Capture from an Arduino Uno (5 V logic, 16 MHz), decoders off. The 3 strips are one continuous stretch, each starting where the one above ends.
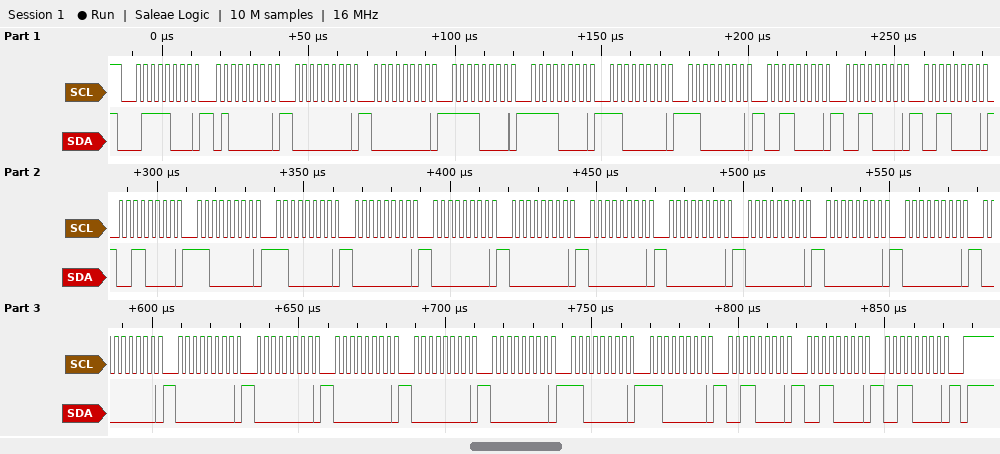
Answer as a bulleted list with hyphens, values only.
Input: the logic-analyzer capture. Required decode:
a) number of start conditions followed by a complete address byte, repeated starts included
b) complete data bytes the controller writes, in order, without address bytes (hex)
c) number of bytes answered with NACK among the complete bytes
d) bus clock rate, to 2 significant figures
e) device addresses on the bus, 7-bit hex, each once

- 1
- 40 00 00 F0 F0 C0 C0 30 30 30 30 C0 C0 00 00 00 00 00 00 00 00 00 00 00 00 00 00 C0 C0 30 30 30
- 0
- 400 kHz
- 0x3C
